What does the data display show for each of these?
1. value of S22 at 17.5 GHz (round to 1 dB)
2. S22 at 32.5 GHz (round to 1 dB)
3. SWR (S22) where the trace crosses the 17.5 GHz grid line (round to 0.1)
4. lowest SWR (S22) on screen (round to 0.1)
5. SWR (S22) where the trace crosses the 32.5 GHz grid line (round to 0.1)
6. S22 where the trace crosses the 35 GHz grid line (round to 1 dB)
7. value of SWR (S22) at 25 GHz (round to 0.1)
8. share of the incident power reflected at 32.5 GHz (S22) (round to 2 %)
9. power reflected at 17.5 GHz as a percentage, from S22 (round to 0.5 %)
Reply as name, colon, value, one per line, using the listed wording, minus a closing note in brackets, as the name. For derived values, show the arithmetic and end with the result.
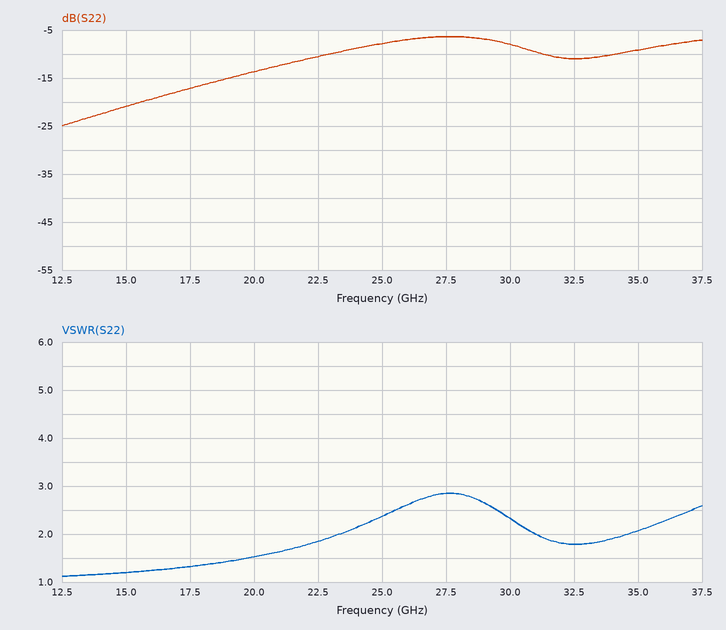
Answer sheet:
value of S22 at 17.5 GHz: -17 dB
S22 at 32.5 GHz: -11 dB
SWR (S22) where the trace crosses the 17.5 GHz grid line: 1.3
lowest SWR (S22) on screen: 1.1
SWR (S22) where the trace crosses the 32.5 GHz grid line: 1.8
S22 where the trace crosses the 35 GHz grid line: -9 dB
value of SWR (S22) at 25 GHz: 2.4
share of the incident power reflected at 32.5 GHz (S22): 10^(-11/10) ≈ 8 %
power reflected at 17.5 GHz as a percentage, from S22: 10^(-17/10) ≈ 2.0 %
